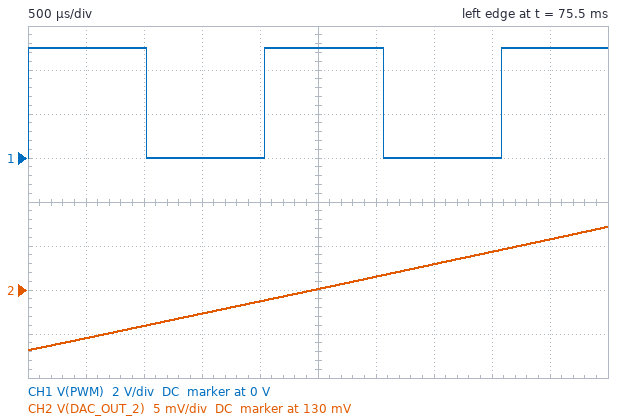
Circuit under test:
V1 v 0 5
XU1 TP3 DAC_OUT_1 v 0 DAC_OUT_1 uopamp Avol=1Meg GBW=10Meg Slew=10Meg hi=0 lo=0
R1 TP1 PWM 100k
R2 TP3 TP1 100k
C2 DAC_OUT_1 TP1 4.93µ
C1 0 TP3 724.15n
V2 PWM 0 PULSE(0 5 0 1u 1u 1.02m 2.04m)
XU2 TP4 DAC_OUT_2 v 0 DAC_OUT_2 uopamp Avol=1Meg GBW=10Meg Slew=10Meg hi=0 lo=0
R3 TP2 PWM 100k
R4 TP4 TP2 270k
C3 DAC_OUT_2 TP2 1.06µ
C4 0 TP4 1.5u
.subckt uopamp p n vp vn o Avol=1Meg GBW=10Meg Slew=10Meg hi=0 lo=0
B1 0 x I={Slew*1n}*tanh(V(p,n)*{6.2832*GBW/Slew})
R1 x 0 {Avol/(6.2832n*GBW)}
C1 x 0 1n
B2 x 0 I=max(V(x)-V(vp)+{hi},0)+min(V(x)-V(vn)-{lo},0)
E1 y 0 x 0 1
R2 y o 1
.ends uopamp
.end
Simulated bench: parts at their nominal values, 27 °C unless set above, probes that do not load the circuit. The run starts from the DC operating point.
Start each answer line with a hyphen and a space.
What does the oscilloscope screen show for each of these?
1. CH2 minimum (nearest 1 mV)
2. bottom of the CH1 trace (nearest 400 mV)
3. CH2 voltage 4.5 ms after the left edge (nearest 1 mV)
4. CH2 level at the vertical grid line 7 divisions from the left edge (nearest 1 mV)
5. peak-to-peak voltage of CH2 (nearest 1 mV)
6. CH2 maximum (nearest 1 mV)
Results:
- 123 mV
- 0 V
- 136 mV
- 133 mV
- 14 mV
- 137 mV
